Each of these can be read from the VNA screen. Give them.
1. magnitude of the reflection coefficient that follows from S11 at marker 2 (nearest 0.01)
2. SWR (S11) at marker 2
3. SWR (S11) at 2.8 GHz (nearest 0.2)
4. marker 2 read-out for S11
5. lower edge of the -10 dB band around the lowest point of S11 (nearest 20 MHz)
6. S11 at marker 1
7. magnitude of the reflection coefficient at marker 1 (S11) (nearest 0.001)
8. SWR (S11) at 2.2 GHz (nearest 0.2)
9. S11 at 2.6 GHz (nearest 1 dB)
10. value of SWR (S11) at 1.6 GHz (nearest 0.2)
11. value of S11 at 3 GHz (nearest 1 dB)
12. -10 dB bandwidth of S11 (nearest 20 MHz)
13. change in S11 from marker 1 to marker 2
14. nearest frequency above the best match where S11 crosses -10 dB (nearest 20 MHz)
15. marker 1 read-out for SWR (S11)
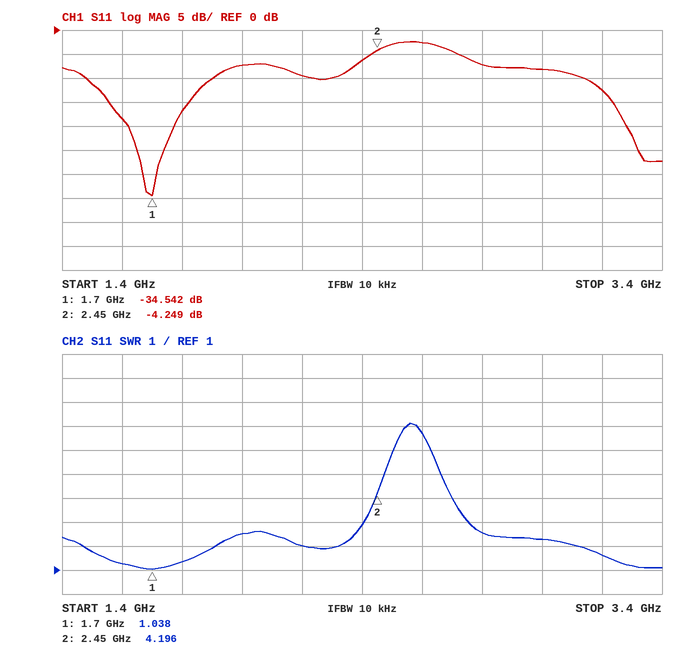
0.61
4.196
2.6
-4.249 dB
1.48 GHz
-34.542 dB
0.019
2.0
-3 dB
1.2
-8 dB
420 MHz
30.293 dB
1.90 GHz
1.038
